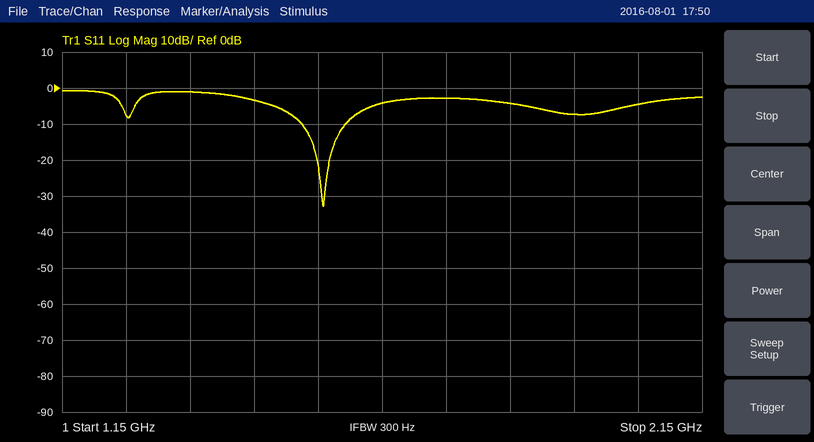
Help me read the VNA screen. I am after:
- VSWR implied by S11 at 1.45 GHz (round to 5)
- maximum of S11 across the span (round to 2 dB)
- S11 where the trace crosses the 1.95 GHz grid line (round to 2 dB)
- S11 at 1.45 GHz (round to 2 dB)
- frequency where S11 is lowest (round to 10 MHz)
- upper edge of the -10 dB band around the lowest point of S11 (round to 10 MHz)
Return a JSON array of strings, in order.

["5", "0 dB", "-8 dB", "-4 dB", "1.56 GHz", "1.59 GHz"]
